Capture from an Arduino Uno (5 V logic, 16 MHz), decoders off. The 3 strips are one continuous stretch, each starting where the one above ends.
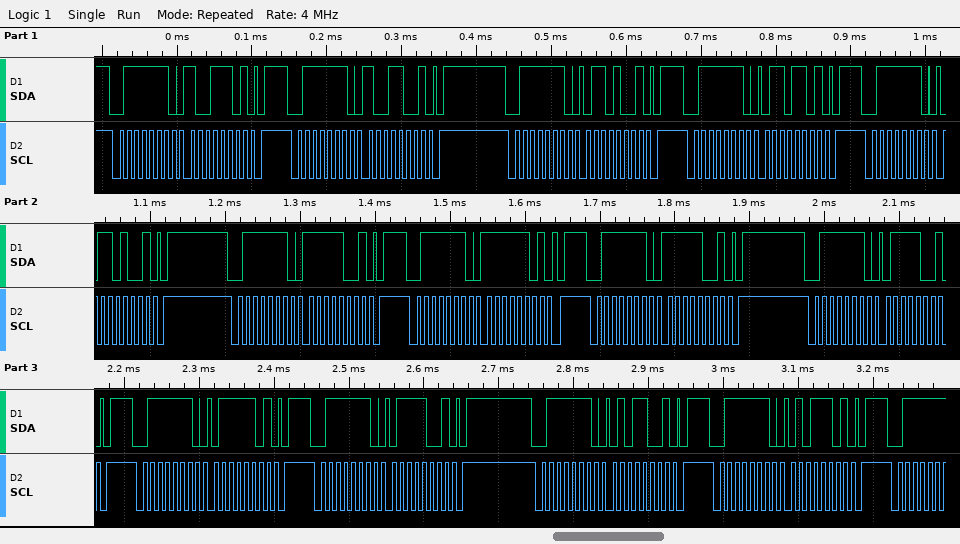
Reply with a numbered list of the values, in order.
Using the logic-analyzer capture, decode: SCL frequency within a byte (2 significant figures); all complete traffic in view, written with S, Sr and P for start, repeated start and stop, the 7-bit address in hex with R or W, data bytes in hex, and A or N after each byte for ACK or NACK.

1. 100 kHz
2. S 3FW A 9D A P S 3FW A 99 A P S 3FW A 69 A P S 3FW A 6D A P S 3FW A 69 A P S 3FW A F9 A P S 3FW A FD A P S 3FW A F9 A P S 3FW A 79 A P S 3FW A 7D A P S 3FW A 79 A P S 3FW A 59 A P S 3FW A 5D A P
